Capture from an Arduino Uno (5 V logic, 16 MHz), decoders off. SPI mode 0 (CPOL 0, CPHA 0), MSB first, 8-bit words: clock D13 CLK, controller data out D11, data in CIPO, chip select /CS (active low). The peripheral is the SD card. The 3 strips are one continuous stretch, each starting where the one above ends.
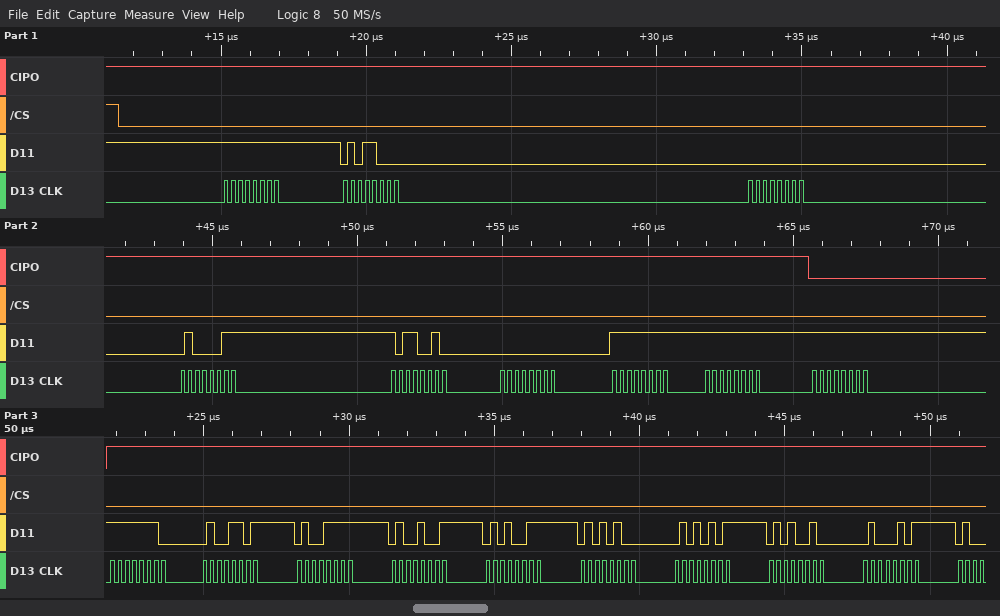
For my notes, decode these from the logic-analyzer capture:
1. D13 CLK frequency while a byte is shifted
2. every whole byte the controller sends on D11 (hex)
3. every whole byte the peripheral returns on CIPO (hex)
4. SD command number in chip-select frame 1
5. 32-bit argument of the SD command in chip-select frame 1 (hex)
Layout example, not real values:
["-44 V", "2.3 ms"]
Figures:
["4 MHz", "FF 58 00 43 B2 00 FF FF FF FE 4D 4F 49 53 54 55 52 45", "FF FF FF FF FF FF FF FF 00 FF FF FF FF FF FF FF FF FF", "CMD24", "0x0043B200"]
